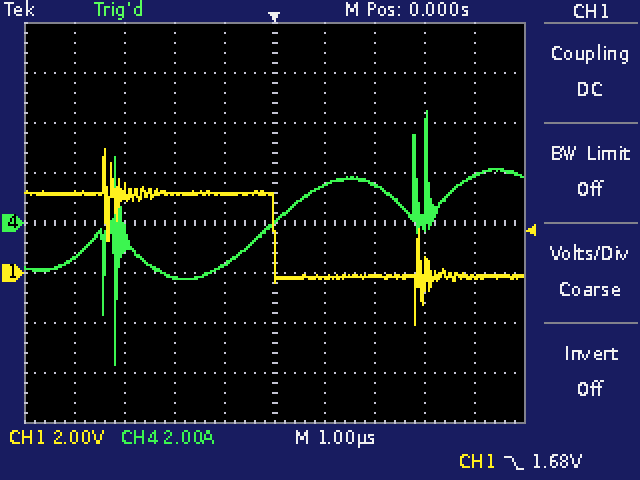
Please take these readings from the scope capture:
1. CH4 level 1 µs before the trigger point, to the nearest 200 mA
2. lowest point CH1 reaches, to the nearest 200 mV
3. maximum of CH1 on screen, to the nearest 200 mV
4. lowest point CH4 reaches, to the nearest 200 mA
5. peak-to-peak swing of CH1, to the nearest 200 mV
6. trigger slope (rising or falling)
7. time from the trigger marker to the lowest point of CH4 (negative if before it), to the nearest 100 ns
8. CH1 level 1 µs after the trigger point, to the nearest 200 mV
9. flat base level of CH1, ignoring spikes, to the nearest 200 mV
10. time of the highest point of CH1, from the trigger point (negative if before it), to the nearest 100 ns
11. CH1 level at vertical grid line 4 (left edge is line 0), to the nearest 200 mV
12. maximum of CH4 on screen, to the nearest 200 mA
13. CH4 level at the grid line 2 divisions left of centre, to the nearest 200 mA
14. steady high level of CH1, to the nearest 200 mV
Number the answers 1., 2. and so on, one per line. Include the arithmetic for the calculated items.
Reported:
1. -1.6 A
2. -2.0 V
3. 5.0 V
4. -5.6 A
5. 5.0 V − (-2.0 V) = 7.0 V
6. falling
7. -3.2 µs
8. -200 mV
9. -200 mV
10. -3.4 µs
11. 3.2 V
12. 4.4 A
13. -2.2 A
14. 3.2 V
